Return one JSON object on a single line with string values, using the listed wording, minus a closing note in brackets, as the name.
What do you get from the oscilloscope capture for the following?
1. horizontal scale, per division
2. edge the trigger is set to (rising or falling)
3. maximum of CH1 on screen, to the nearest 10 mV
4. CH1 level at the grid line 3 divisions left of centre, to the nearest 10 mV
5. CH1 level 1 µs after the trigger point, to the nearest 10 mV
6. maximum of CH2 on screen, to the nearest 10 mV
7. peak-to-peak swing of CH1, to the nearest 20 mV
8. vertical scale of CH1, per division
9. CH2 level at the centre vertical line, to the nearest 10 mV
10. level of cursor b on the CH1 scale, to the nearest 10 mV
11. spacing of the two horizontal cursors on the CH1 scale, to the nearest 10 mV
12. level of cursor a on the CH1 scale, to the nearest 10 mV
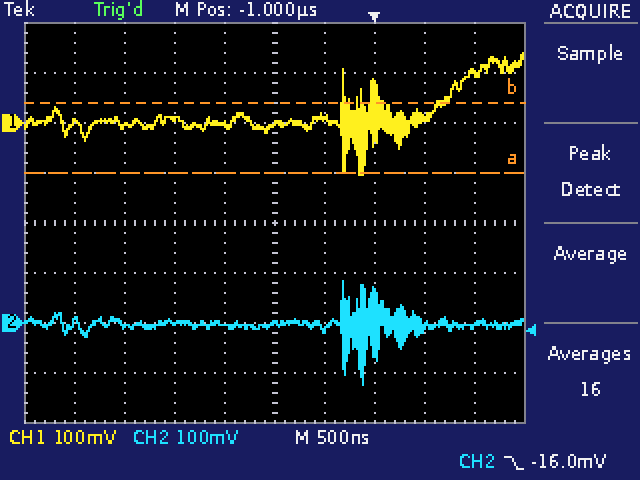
{"horizontal scale, per division": "500 ns", "edge the trigger is set to": "falling", "maximum of CH1 on screen, to the nearest 10 mV": "140 mV", "CH1 level at the grid line 3 divisions left of centre, to the nearest 10 mV": "-10 mV", "CH1 level 1 µs after the trigger point, to the nearest 10 mV": "100 mV", "maximum of CH2 on screen, to the nearest 10 mV": "80 mV", "peak-to-peak swing of CH1, to the nearest 20 mV": "240 mV", "vertical scale of CH1, per division": "100 mV", "CH2 level at the centre vertical line, to the nearest 10 mV": "0 mV", "level of cursor b on the CH1 scale, to the nearest 10 mV": "40 mV", "spacing of the two horizontal cursors on the CH1 scale, to the nearest 10 mV": "140 mV", "level of cursor a on the CH1 scale, to the nearest 10 mV": "-100 mV"}
